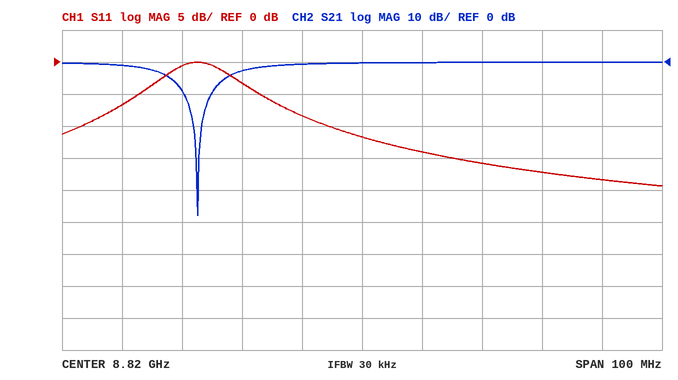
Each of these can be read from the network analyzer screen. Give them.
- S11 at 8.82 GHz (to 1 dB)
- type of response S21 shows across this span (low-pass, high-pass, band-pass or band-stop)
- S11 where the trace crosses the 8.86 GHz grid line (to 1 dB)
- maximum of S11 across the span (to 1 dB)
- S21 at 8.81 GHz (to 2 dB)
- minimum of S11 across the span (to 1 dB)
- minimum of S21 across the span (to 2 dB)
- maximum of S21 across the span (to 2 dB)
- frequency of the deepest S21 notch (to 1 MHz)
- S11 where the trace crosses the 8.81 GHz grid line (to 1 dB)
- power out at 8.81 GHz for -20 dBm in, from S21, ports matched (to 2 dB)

-12 dB
band-stop
-18 dB
0 dB
0 dB
-19 dB
-48 dB
0 dB
8.793 GHz
-8 dB
-20 dBm
